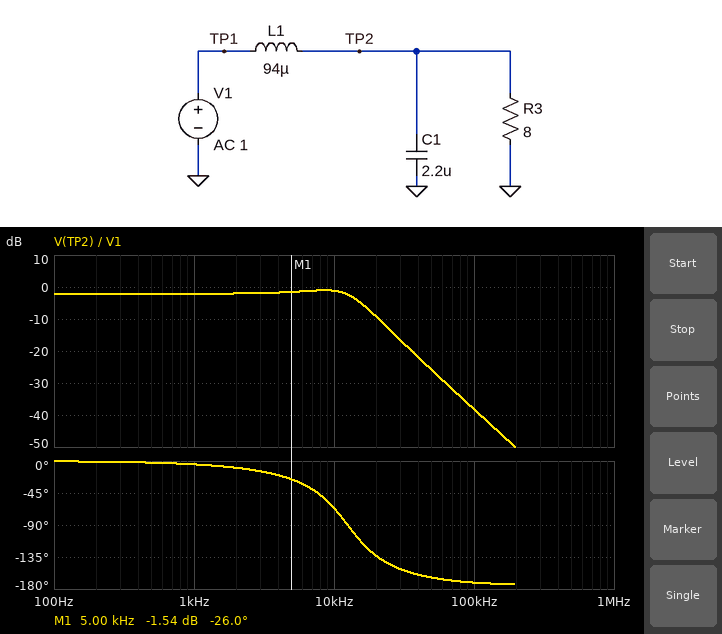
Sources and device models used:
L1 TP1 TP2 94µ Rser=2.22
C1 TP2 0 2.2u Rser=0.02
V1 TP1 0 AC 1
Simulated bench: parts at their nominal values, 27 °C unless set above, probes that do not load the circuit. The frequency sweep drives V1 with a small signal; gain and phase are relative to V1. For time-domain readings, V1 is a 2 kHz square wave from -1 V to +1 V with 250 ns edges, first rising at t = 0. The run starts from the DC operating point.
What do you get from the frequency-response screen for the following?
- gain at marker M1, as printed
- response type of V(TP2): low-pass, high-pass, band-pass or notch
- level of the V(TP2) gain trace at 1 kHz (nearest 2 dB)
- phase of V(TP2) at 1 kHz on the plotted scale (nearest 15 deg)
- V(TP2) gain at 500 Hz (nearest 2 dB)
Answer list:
-1.54 dB
low-pass
-2 dB
0 deg
-2 dB
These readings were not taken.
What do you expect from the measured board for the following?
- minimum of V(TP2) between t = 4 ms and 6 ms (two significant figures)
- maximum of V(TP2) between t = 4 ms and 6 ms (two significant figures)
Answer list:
-1.0 V
1.0 V
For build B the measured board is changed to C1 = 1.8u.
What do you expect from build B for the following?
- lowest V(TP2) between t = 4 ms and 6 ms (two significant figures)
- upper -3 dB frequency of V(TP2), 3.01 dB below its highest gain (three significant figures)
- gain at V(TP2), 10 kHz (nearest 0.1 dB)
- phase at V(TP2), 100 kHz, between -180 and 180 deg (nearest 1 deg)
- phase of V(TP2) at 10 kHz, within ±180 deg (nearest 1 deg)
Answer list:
-1.0 V
15.9 kHz
-1.3 dB
-170 deg
-58 deg
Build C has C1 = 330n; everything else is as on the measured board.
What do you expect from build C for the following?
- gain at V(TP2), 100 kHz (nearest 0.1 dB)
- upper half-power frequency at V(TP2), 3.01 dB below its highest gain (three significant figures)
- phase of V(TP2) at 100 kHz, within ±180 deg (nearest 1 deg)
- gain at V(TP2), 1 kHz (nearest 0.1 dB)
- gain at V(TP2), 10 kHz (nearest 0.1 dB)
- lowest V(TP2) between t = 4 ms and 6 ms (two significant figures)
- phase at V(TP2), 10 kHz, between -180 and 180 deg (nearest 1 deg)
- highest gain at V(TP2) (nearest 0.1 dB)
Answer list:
-22.6 dB
21.0 kHz
-144 deg
-2.1 dB
-2.9 dB
-780 mV
-34 deg
-2.1 dB
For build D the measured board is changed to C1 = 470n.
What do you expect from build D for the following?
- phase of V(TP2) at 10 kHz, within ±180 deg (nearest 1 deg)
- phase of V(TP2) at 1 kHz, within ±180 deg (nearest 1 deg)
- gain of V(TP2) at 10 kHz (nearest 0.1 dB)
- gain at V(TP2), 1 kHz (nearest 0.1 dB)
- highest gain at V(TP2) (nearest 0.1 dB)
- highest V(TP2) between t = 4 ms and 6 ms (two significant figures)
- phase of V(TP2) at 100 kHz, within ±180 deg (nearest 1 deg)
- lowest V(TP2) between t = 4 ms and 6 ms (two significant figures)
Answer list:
-36 deg
-4 deg
-2.7 dB
-2.1 dB
-2.1 dB
790 mV
-153 deg
-790 mV
